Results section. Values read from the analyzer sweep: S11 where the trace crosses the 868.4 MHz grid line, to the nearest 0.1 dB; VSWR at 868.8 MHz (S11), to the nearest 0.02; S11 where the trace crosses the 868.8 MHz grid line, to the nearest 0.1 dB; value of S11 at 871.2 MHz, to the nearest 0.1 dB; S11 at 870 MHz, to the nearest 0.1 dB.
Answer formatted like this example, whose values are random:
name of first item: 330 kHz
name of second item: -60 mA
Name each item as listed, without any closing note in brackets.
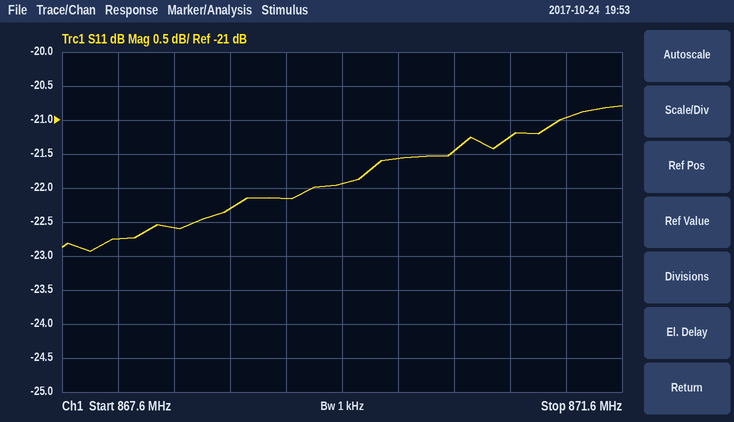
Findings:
S11 where the trace crosses the 868.4 MHz grid line, to the nearest 0.1 dB: -22.6 dB
VSWR at 868.8 MHz (S11), to the nearest 0.02: 1.16
S11 where the trace crosses the 868.8 MHz grid line, to the nearest 0.1 dB: -22.3 dB
value of S11 at 871.2 MHz, to the nearest 0.1 dB: -21.0 dB
S11 at 870 MHz, to the nearest 0.1 dB: -21.6 dB
